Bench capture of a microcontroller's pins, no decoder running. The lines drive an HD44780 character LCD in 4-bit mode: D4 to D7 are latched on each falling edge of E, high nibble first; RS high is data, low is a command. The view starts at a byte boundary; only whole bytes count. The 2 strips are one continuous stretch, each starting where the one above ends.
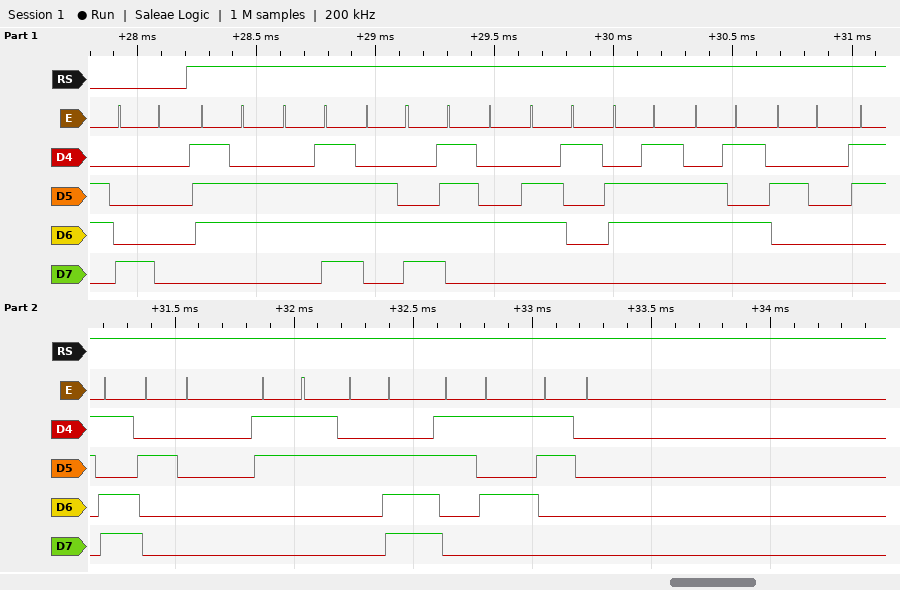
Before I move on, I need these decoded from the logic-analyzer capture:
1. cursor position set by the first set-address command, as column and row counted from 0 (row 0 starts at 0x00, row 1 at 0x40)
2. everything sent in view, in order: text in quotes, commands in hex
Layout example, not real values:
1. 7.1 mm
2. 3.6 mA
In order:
1. column 0, row 0
2. 0x80 "voltage = 3.50"
